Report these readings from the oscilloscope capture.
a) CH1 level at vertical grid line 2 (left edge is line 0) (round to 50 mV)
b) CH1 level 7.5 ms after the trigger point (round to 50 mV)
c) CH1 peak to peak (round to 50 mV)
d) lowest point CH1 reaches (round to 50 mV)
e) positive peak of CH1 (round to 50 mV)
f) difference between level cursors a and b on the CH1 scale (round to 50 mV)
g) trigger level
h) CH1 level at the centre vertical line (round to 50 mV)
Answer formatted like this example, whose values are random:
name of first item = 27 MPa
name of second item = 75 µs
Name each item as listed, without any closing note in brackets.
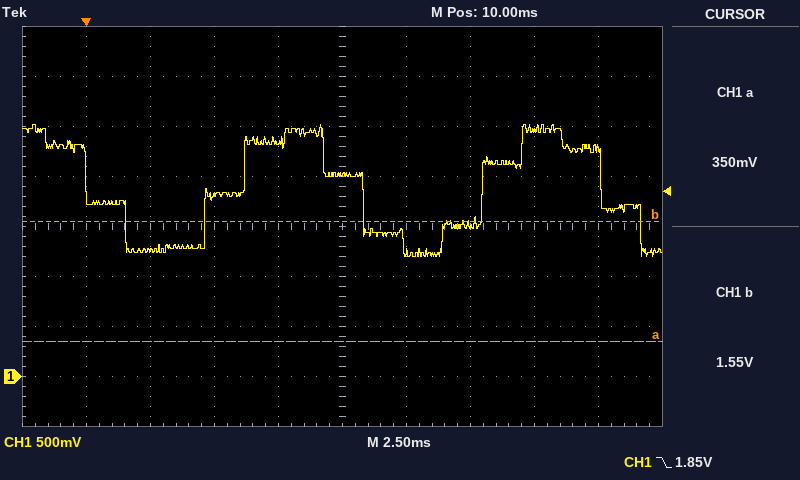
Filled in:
CH1 level at vertical grid line 2 (left edge is line 0) = 1.25 V
CH1 level 7.5 ms after the trigger point = 2.35 V
CH1 peak to peak = 1.30 V
lowest point CH1 reaches = 1.20 V
positive peak of CH1 = 2.50 V
difference between level cursors a and b on the CH1 scale = 1.20 V
trigger level = 1.85 V
CH1 level at the centre vertical line = 2.00 V
